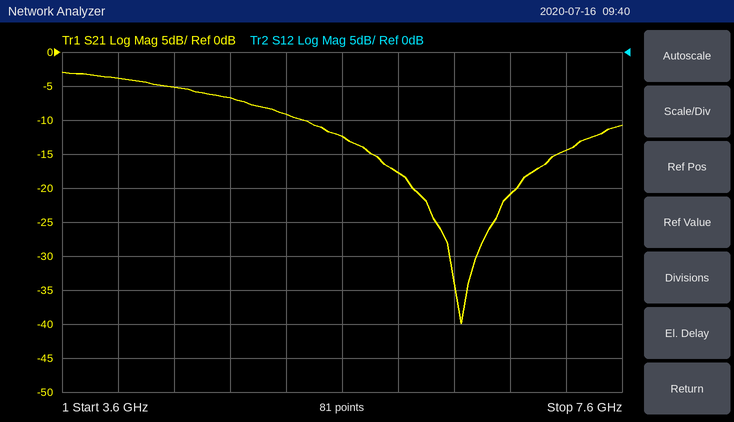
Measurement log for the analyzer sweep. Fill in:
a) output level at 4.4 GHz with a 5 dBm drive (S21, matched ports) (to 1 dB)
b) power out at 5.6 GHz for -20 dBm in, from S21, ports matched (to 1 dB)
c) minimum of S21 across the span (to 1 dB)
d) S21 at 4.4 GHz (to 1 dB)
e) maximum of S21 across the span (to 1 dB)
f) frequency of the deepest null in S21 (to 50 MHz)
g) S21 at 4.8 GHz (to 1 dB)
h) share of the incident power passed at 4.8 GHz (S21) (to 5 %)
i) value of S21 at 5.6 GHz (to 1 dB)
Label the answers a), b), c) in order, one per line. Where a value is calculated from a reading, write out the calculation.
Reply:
a) 5 dBm + (-5 dB) = 0 dBm
b) -20 dBm + (-12 dB) = -32 dBm
c) -40 dB
d) -5 dB
e) -3 dB
f) 6.45 GHz
g) -7 dB
h) 10^(-7/10) ≈ 20 %
i) -12 dB
